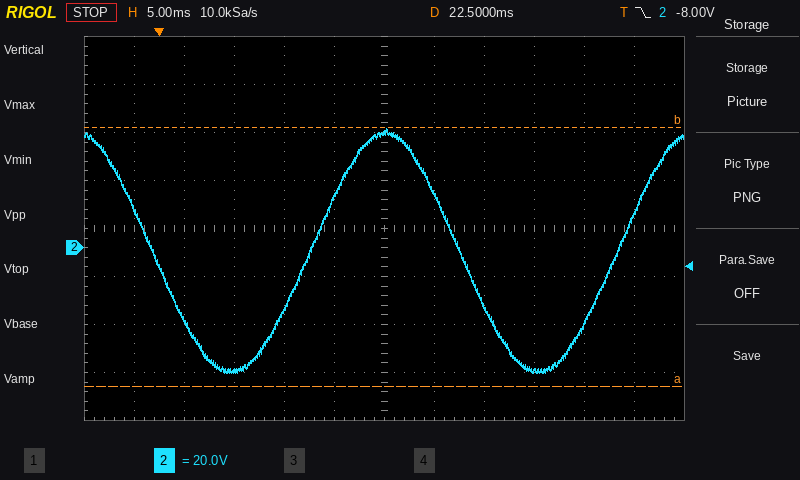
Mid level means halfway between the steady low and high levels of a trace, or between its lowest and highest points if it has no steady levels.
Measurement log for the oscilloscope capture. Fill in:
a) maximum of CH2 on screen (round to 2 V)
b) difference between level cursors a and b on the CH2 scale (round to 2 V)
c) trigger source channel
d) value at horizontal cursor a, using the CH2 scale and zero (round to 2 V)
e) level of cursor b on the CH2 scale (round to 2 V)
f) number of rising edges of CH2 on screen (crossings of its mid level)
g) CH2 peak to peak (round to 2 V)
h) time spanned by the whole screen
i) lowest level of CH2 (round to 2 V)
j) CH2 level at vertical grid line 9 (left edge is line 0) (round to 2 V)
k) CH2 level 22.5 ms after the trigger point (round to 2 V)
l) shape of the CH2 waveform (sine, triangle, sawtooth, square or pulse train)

50 V
108 V
CH2
-58 V
50 V
2
102 V
60 ms
-52 V
-52 V
48 V
sine
